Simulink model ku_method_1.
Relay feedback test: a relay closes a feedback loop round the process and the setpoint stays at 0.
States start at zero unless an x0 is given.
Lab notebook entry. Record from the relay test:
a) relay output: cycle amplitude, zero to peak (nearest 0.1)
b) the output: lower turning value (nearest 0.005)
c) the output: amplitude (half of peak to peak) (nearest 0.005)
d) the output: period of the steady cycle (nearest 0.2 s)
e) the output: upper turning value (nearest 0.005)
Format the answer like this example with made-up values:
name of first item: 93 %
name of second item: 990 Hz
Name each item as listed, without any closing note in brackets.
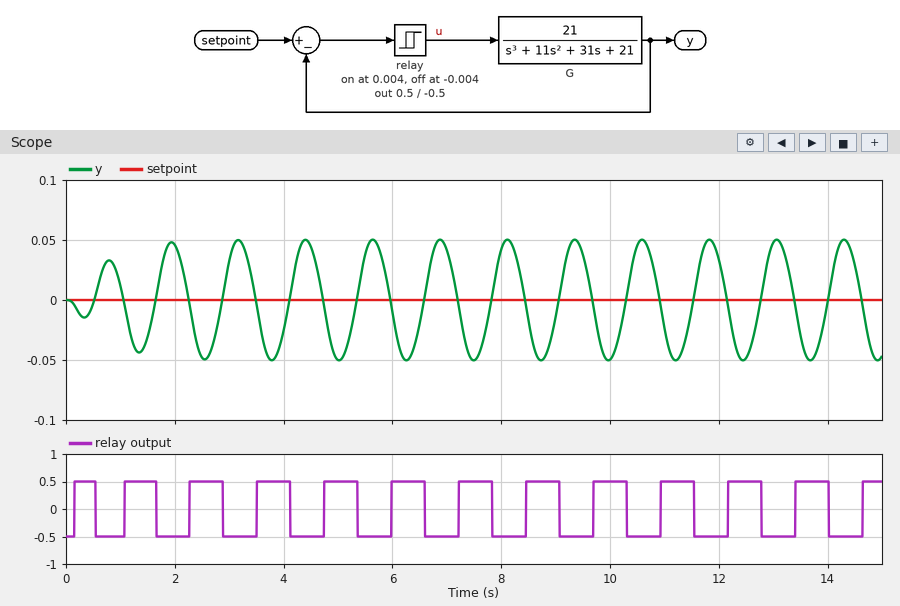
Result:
relay output: cycle amplitude, zero to peak: 0.5
the output: lower turning value: -0.050
the output: amplitude (half of peak to peak): 0.050
the output: period of the steady cycle: 1.2 s
the output: upper turning value: 0.050
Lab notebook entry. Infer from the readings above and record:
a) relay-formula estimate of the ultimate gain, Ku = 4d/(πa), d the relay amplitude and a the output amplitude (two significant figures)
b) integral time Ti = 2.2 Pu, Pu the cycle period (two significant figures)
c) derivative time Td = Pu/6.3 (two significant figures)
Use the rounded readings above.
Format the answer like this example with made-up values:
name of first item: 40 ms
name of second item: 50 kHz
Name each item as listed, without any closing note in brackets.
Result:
relay-formula estimate of the ultimate gain, Ku = 4d/(πa), d the relay amplitude and a the output amplitude: 13
integral time Ti = 2.2 Pu, Pu the cycle period: 2.6 s
derivative time Td = Pu/6.3: 0.19 s
